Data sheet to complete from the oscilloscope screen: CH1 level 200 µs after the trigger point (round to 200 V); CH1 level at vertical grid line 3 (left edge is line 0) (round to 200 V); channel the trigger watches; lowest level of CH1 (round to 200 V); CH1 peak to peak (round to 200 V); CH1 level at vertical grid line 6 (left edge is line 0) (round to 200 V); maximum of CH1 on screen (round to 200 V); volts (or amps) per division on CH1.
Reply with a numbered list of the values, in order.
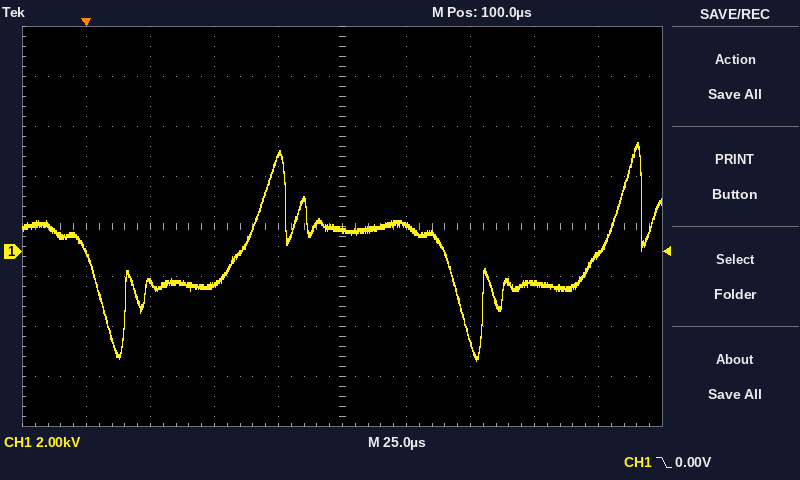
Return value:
1. -200 V
2. -1.4 kV
3. CH1
4. -4.4 kV
5. 8.8 kV
6. 1.0 kV
7. 4.4 kV
8. 2 kV
